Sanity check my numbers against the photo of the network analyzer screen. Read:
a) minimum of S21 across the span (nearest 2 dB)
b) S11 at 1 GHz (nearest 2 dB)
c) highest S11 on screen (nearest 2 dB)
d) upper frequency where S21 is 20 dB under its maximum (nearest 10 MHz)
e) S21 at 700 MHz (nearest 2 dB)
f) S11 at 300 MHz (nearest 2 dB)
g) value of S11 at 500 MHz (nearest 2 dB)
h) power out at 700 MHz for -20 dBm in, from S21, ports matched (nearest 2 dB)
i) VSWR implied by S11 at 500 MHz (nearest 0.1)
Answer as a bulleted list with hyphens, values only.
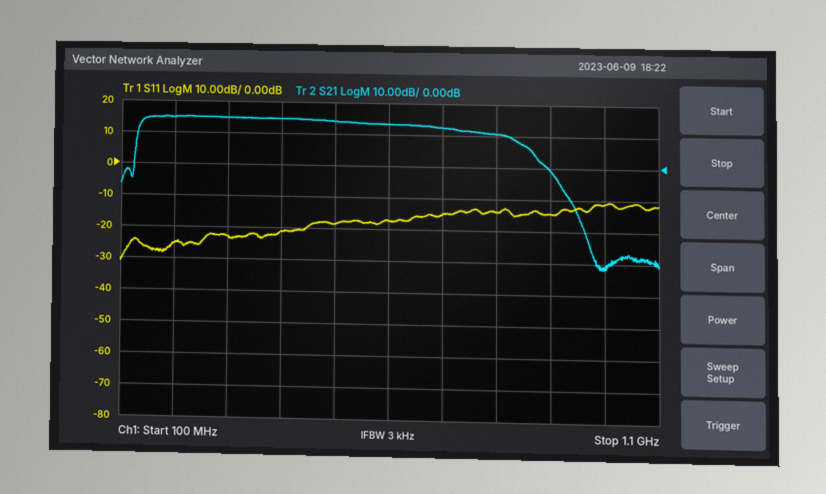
- -32 dB
- -12 dB
- -10 dB
- 920 MHz
- 12 dB
- -22 dB
- -18 dB
- -8 dBm
- 1.3
